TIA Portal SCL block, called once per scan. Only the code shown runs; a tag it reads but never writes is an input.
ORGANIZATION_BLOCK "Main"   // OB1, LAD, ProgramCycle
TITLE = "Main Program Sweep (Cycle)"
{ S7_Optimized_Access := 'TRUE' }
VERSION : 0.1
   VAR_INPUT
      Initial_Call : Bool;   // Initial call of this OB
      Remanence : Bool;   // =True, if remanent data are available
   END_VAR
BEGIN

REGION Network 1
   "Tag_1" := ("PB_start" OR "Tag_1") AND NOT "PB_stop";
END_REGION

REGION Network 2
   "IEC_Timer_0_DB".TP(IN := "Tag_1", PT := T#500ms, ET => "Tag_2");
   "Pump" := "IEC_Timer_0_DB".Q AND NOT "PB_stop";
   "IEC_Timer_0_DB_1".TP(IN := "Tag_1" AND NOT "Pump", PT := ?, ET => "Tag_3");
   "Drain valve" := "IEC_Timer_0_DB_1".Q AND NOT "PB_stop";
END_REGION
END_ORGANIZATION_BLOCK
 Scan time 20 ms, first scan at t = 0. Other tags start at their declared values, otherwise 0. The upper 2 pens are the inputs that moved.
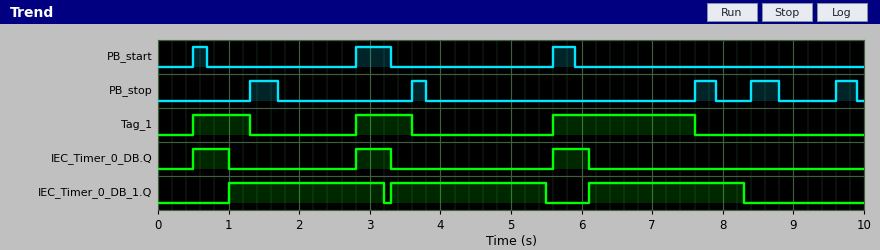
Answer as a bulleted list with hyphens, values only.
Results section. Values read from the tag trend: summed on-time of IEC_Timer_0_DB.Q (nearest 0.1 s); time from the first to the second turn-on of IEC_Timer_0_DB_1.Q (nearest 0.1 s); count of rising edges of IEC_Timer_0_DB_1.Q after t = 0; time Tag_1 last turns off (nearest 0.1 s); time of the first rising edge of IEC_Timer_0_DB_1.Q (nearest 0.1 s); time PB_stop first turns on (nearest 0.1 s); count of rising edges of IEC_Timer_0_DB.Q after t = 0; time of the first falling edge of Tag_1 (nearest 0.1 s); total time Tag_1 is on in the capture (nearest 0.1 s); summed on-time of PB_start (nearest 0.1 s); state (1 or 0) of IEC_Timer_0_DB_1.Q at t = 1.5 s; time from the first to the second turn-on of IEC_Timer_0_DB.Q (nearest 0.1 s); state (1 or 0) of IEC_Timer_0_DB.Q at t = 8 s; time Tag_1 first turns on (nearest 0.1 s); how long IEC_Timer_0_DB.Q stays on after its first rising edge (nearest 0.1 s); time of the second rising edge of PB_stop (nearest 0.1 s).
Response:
- 1.5 s
- 2.3 s
- 3
- 7.6 s
- 1.0 s
- 1.3 s
- 3
- 1.3 s
- 3.6 s
- 1.0 s
- 1
- 2.3 s
- 0
- 0.5 s
- 0.5 s
- 3.6 s
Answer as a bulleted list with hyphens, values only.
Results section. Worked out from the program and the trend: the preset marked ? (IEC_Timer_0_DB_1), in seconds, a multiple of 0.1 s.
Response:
- 2.2 s
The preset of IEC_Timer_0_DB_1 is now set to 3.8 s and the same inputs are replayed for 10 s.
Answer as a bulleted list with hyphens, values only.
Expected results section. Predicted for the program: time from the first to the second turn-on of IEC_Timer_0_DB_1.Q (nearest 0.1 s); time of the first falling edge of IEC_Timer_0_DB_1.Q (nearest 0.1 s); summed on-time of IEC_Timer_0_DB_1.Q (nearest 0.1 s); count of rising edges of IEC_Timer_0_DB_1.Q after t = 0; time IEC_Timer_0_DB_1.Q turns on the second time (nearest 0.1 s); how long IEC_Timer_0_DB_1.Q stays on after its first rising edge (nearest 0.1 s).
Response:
- 5.1 s
- 4.8 s
- 7.6 s
- 2
- 6.1 s
- 3.8 s
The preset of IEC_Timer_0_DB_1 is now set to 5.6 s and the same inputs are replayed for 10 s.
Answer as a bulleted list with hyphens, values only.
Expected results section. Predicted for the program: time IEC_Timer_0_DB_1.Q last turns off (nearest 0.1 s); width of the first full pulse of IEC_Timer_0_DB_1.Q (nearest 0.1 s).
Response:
- 6.6 s
- 5.6 s
